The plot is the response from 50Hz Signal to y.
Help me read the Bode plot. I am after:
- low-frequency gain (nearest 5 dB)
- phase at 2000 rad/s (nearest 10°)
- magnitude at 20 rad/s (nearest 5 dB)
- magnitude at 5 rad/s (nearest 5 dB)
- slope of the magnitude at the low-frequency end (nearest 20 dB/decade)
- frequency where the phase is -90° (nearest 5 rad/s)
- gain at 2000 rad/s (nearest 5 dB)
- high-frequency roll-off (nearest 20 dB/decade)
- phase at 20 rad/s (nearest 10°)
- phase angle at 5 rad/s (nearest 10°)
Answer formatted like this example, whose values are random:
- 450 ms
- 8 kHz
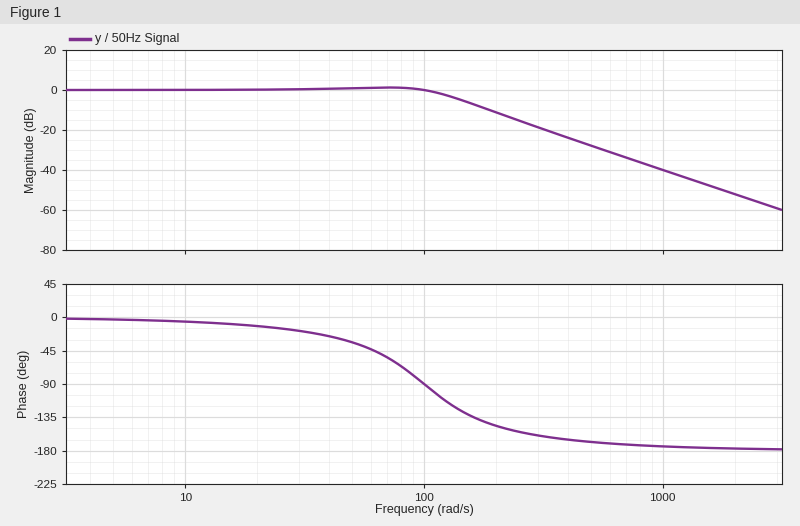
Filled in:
- 0 dB
- -180°
- 0 dB
- 0 dB
- 0 dB/decade
- 100 rad/s
- -50 dB
- -40 dB/decade
- -10°
- 0°
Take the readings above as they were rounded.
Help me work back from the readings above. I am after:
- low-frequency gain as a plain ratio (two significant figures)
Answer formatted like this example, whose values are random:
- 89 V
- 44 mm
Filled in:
- 1.0
